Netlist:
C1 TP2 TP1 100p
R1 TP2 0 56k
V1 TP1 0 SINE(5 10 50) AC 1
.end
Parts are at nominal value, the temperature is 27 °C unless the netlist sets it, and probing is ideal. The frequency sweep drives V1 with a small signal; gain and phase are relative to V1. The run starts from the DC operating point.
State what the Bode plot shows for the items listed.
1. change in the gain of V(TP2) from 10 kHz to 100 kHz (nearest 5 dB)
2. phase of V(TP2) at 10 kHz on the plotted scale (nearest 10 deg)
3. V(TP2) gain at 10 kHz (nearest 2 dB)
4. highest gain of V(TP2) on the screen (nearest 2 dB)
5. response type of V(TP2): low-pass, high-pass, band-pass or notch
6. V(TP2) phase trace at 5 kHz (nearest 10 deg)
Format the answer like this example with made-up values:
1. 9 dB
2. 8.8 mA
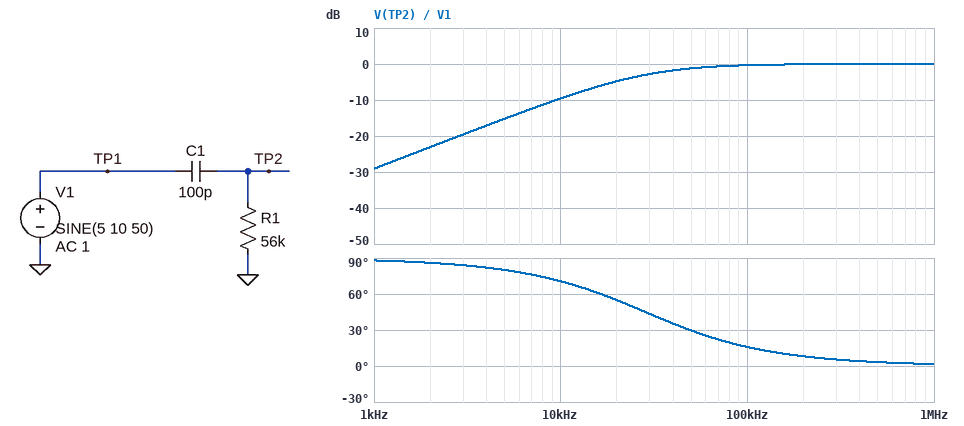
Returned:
1. 10 dB
2. 70 deg
3. -10 dB
4. 0 dB
5. high-pass
6. 80 deg
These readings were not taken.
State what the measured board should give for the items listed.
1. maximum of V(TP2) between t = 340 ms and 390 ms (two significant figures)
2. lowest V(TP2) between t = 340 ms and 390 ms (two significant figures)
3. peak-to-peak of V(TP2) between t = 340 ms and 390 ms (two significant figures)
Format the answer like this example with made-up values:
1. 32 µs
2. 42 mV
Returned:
1. 18 mV
2. -18 mV
3. 35 mV
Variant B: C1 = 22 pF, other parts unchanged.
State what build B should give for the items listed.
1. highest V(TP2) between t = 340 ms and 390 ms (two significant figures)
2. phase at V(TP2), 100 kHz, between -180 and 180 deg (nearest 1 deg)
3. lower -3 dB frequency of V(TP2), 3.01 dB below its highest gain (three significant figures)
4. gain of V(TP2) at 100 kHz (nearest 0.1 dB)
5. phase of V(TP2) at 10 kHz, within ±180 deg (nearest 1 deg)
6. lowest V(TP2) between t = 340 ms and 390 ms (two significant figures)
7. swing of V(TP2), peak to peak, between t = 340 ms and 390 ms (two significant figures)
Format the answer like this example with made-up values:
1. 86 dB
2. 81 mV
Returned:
1. 3.9 mV
2. 52 deg
3. 129 kHz
4. -4.3 dB
5. 86 deg
6. -3.9 mV
7. 7.7 mV
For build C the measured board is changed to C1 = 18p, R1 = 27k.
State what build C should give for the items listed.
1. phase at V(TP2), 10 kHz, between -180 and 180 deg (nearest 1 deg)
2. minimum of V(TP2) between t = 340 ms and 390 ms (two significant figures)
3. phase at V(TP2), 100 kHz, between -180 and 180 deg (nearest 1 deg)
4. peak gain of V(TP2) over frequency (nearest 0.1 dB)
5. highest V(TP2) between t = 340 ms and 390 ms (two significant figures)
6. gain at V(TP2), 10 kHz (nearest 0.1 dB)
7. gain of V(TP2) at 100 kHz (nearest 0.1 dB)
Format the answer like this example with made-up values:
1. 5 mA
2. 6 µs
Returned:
1. 88 deg
2. -1.5 mV
3. 73 deg
4. 0 dB
5. 1.5 mV
6. -30.3 dB
7. -10.7 dB
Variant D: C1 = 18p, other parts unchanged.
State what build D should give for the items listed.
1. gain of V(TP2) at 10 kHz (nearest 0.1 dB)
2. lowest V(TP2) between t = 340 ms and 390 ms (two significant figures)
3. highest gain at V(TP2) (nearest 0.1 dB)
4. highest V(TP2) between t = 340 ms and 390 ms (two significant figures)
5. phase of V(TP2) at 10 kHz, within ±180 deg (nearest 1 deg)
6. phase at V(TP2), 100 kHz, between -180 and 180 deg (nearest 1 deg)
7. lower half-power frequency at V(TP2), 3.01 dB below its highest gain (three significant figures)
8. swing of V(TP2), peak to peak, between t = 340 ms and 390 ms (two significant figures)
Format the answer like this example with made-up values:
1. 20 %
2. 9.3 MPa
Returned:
1. -24.0 dB
2. -3.2 mV
3. 0 dB
4. 3.2 mV
5. 86 deg
6. 58 deg
7. 158 kHz
8. 6.3 mV
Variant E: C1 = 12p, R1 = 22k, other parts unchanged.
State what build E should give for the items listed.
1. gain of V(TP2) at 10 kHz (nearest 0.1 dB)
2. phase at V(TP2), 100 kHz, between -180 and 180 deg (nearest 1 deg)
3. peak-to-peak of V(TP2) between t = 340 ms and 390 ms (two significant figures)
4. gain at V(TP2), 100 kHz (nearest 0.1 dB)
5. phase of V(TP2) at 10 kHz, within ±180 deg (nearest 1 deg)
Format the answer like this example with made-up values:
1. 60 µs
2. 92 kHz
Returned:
1. -35.6 dB
2. 81 deg
3. 1.7 mV
4. -15.7 dB
5. 89 deg
